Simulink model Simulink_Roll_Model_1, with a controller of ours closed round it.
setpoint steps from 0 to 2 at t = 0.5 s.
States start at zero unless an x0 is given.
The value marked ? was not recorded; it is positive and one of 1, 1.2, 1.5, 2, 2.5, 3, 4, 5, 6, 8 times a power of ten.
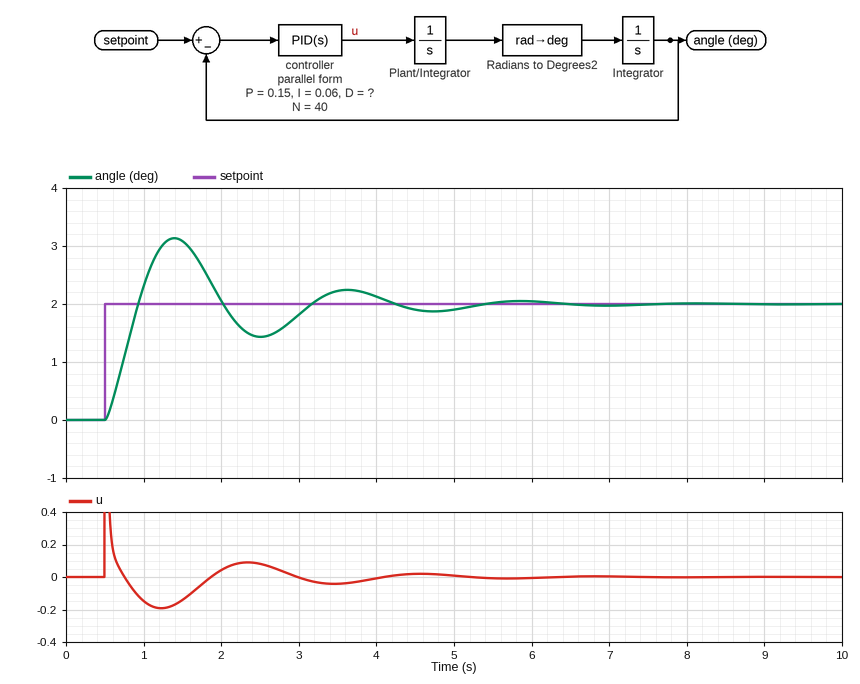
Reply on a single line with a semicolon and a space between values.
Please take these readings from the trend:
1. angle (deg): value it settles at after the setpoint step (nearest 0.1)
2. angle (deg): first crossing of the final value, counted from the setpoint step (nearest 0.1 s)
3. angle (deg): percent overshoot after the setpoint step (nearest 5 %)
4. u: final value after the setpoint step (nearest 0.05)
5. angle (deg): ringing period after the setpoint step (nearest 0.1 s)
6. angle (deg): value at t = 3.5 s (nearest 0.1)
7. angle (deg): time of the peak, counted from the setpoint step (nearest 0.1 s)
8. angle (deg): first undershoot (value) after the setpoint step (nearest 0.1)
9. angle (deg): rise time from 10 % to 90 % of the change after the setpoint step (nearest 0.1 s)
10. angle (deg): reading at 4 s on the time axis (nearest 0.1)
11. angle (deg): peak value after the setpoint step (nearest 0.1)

2.0; 0.4 s; 55 %; 0.00; 2.2 s; 2.2; 0.9 s; 1.4; 0.3 s; 2.1; 3.1
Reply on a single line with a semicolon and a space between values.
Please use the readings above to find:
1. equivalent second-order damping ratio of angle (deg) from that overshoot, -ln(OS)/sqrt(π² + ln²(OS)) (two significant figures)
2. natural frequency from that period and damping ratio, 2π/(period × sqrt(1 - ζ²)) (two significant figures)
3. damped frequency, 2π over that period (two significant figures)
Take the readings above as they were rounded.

0.19; 2.9 rad/s; 2.9 rad/s
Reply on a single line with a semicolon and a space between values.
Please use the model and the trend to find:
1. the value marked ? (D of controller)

0.03
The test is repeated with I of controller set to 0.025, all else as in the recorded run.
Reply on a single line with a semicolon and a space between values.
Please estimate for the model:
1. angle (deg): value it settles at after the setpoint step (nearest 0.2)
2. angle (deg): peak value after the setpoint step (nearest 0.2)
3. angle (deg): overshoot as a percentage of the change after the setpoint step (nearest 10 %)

2.0; 3.0; 50 %
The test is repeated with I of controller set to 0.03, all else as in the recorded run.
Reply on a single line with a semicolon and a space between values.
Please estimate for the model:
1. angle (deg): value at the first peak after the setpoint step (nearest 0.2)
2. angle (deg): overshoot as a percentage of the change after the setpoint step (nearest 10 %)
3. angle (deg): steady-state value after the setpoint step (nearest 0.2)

3.0; 50 %; 2.0
